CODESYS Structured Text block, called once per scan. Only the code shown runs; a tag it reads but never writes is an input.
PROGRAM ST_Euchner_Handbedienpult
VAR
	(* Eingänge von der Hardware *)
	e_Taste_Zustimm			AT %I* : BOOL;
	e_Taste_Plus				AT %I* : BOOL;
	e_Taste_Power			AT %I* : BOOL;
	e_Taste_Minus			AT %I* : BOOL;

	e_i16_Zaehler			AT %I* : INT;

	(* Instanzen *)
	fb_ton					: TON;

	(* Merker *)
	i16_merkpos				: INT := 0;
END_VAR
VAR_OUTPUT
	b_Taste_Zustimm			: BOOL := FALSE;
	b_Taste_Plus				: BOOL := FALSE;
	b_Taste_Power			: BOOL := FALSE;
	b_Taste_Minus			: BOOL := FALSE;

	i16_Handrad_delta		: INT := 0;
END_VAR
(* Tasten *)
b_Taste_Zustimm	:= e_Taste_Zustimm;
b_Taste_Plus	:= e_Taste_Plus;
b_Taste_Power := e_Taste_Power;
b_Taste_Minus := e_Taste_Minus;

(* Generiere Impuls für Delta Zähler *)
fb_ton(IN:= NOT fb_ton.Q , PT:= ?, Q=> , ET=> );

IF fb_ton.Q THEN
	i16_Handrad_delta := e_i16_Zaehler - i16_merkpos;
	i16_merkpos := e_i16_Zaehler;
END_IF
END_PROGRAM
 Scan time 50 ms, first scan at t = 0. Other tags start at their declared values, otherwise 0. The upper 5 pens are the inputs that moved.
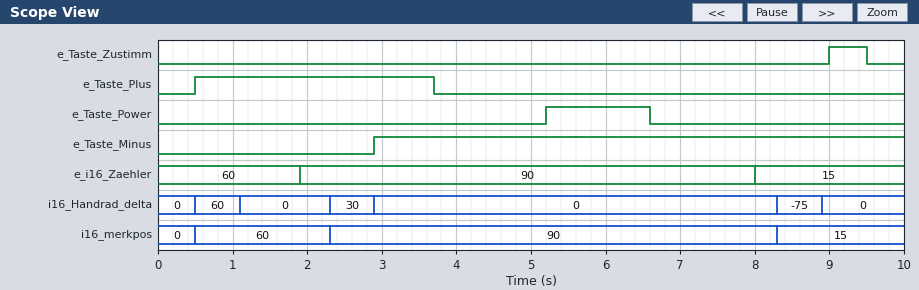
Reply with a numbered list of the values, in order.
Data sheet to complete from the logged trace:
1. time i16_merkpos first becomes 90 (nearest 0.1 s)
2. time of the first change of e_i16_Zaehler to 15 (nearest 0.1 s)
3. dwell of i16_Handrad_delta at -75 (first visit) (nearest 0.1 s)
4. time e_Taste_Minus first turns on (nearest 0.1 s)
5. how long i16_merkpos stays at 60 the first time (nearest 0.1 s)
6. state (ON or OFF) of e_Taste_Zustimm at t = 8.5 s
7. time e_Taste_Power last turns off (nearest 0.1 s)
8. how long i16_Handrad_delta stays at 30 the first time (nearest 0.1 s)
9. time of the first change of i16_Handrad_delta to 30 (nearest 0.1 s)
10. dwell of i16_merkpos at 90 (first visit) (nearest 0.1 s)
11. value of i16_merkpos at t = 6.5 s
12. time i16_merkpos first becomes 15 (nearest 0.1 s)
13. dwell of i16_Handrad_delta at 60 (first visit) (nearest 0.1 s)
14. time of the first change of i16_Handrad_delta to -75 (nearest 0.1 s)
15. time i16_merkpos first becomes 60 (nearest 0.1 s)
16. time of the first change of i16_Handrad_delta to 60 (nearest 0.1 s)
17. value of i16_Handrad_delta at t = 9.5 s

1. 2.3 s
2. 8.0 s
3. 0.6 s
4. 2.9 s
5. 1.8 s
6. OFF
7. 6.6 s
8. 0.6 s
9. 2.3 s
10. 6.0 s
11. 90
12. 8.3 s
13. 0.6 s
14. 8.3 s
15. 0.5 s
16. 0.5 s
17. 0
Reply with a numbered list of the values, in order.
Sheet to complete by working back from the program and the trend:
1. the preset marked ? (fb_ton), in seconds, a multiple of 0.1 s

1. 0.5 s
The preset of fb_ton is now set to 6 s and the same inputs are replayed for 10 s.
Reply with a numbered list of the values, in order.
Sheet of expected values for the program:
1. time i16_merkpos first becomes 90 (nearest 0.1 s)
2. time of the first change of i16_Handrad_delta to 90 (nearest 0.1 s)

1. 6.0 s
2. 6.0 s
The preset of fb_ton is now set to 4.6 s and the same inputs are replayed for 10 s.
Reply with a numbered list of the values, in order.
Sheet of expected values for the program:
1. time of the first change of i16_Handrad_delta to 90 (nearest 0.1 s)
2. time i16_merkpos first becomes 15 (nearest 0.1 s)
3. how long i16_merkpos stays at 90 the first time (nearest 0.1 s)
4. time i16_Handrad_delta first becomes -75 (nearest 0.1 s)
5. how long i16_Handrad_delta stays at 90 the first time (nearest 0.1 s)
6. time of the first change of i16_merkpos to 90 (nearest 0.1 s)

1. 4.6 s
2. 9.3 s
3. 4.7 s
4. 9.3 s
5. 4.7 s
6. 4.6 s
